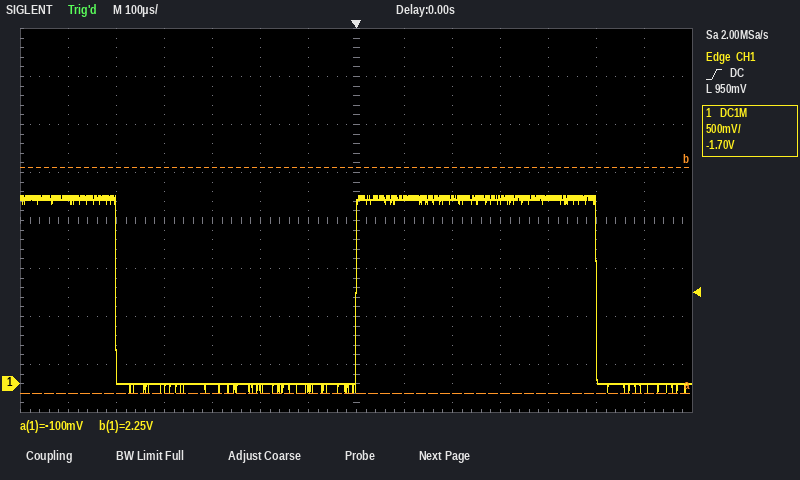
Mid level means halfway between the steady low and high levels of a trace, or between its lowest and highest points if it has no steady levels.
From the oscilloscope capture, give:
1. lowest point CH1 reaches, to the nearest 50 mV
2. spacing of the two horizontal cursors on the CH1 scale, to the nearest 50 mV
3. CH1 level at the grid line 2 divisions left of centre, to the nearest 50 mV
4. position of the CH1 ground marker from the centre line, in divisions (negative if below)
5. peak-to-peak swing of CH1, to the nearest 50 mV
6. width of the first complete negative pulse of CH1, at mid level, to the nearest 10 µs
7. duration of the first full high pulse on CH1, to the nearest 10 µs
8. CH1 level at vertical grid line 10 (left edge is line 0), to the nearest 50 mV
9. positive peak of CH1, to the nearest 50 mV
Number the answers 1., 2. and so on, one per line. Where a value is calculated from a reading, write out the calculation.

1. -100 mV
2. 2.35 V
3. -50 mV
4. -3.4 div
5. 1.95 V − (-100 mV) = 2.05 V
6. 500 µs
7. 500 µs
8. 1.90 V
9. 1.95 V
